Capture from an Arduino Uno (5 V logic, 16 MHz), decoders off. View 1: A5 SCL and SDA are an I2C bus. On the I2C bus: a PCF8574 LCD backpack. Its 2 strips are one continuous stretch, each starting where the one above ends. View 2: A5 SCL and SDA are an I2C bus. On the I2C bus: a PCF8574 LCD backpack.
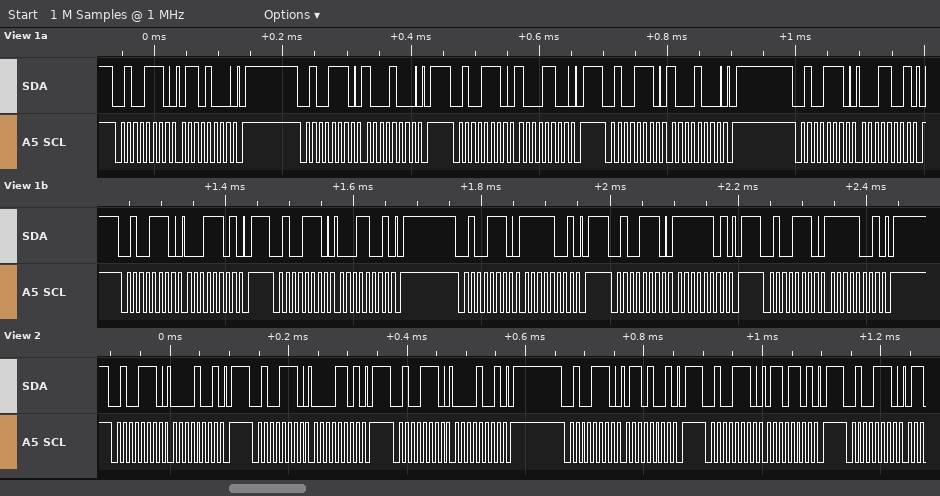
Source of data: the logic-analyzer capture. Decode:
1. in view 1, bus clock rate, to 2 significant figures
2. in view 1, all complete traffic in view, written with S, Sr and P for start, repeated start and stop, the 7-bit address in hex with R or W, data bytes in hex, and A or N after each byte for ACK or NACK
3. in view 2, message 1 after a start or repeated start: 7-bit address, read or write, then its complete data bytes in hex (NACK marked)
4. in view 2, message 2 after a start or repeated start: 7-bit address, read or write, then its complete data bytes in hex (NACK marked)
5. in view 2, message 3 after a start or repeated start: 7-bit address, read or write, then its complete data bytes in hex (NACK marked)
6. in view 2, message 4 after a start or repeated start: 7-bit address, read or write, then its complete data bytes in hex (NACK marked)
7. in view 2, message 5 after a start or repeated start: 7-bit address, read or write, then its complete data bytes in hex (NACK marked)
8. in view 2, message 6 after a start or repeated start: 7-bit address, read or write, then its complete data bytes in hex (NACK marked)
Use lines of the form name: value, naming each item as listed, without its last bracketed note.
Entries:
in view 1, bus clock rate, to 2 significant figures: 100 kHz
in view 1, all complete traffic in view, written with S, Sr and P for start, repeated start and stop, the 7-bit address in hex with R or W, data bytes in hex, and A or N after each byte for ACK or NACK: S 27W A 68 A P S 27W A 88 A P S 27W A 8C A P S 27W A 88 A P S 27W A 19 A P S 27W A 1D A P S 27W A 19 A P S 27W A F9 A P S 27W A FD A P S 27W A F9 A P
in view 2, message 1 after a start or repeated start: 7-bit address, read or write, then its complete data bytes in hex: 0x27 write: 09
in view 2, message 2 after a start or repeated start: 7-bit address, read or write, then its complete data bytes in hex: 0x27 write: 0D
in view 2, message 3 after a start or repeated start: 7-bit address, read or write, then its complete data bytes in hex: 0x27 write: 09
in view 2, message 4 after a start or repeated start: 7-bit address, read or write, then its complete data bytes in hex: 0x27 write: 69
in view 2, message 5 after a start or repeated start: 7-bit address, read or write, then its complete data bytes in hex: 0x27 write: 6D
in view 2, message 6 after a start or repeated start: 7-bit address, read or write, then its complete data bytes in hex: 0x27 write
